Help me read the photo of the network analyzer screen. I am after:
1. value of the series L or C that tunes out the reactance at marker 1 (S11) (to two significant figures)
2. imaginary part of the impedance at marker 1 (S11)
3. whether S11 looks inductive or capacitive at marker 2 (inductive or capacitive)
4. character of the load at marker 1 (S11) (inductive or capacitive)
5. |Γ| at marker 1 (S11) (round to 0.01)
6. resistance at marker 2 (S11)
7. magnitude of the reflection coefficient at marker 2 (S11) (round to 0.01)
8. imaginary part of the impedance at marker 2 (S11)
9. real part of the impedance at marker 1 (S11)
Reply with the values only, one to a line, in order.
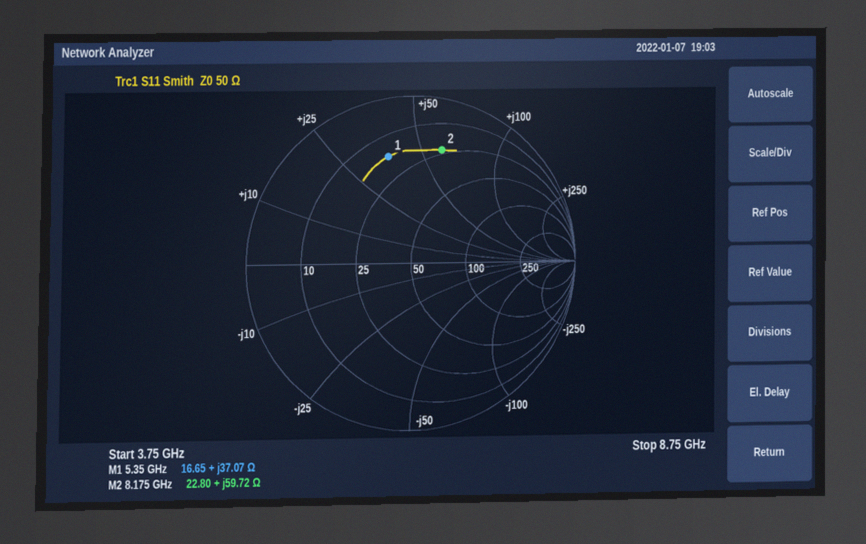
800 fF
+37.07 Ω
inductive
inductive
0.65
22.80 Ω
0.70
+59.72 Ω
16.65 Ω
